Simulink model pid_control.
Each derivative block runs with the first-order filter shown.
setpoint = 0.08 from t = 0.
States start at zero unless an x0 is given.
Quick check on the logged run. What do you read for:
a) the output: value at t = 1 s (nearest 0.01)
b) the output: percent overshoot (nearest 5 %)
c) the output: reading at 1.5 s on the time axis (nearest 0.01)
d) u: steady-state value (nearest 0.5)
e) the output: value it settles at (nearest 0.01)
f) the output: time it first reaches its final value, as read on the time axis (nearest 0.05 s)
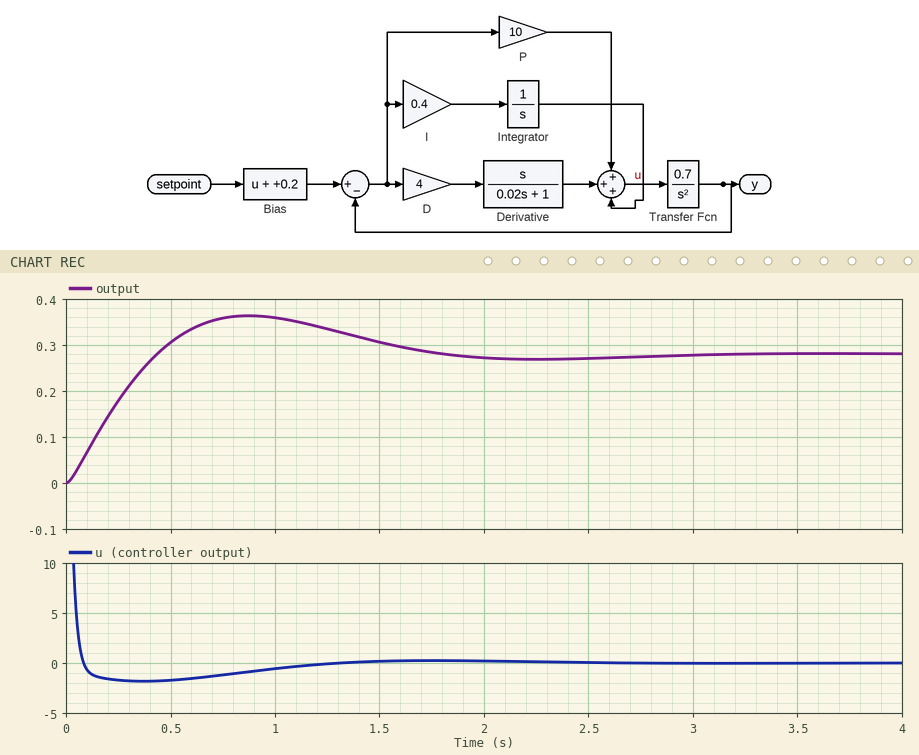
0.36
30 %
0.31
0.0
0.28
0.45 s
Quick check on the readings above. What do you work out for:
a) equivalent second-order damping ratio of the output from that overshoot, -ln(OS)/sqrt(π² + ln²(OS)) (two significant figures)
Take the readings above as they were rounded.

0.36
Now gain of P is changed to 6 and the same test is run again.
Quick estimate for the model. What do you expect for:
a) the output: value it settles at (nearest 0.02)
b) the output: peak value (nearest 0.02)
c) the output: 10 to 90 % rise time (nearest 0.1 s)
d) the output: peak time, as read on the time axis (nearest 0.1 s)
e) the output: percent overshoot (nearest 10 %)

0.28
0.34
0.4 s
1.1 s
20 %
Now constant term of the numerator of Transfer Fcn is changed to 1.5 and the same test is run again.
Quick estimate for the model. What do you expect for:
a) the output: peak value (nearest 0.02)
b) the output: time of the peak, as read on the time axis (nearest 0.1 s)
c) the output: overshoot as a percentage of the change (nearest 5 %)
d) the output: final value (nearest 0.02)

0.34
0.5 s
20 %
0.28
